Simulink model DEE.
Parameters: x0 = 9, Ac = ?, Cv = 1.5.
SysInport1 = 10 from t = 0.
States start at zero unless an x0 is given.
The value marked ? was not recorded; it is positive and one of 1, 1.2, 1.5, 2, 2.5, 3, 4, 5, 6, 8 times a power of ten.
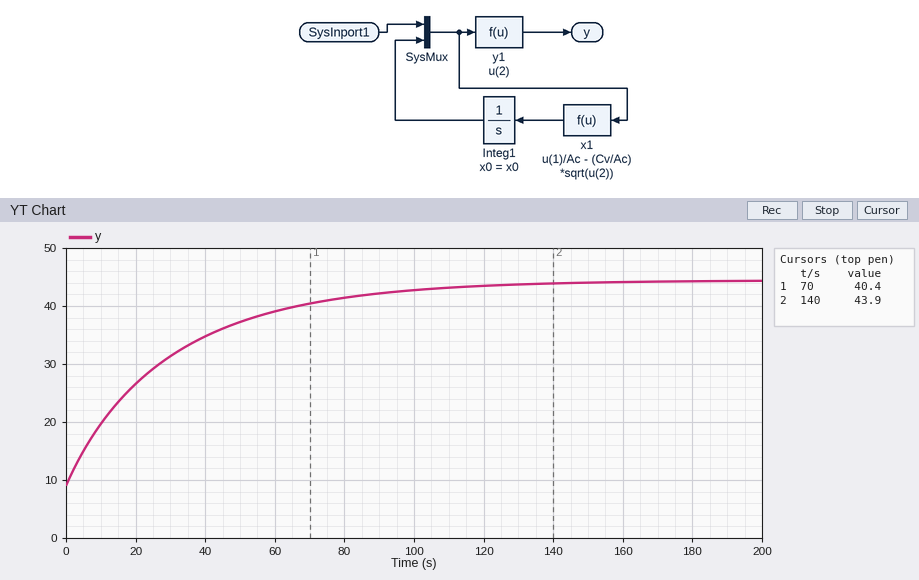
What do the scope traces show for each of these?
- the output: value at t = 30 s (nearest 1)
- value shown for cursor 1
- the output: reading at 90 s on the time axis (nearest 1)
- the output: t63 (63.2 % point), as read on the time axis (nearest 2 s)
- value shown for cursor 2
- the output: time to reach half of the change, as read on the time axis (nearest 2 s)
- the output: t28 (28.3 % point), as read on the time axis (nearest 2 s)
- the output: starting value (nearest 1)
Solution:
31
40.4
42
30 s
43.9
20 s
10 s
9
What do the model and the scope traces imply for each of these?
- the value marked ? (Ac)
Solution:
4
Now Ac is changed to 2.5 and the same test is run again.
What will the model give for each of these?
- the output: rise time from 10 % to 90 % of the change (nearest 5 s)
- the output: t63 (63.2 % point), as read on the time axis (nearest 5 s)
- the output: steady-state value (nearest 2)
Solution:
45 s
20 s
44
